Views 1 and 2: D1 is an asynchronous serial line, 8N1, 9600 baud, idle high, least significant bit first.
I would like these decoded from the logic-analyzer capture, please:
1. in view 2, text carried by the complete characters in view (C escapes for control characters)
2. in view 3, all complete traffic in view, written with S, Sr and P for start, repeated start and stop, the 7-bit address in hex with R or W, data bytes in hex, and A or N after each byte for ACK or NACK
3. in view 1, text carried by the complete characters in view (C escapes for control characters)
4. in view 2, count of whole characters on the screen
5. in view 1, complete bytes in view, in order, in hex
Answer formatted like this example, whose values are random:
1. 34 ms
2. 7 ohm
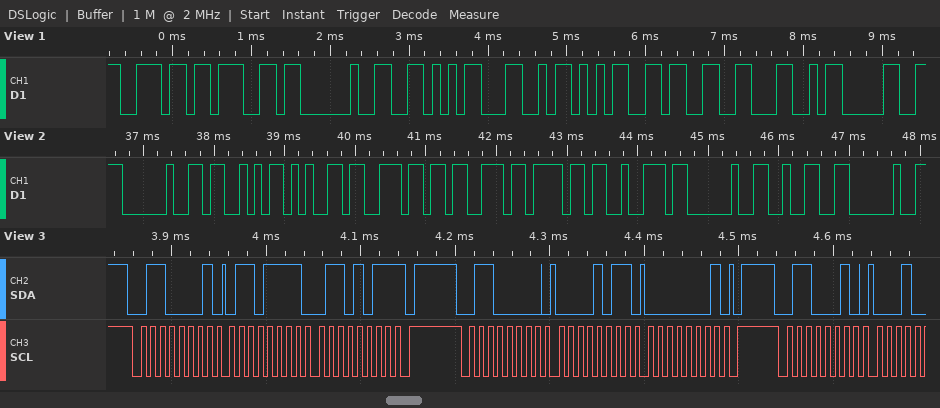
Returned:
1. " Sensor 2 "
2. S 30R A 6F A 6B N P S 30W A 0B A 01 A P S 31W A
3. "ng VL53L0"
4. 10
5. 6E 67 20 56 4C 35 33 4C 30
